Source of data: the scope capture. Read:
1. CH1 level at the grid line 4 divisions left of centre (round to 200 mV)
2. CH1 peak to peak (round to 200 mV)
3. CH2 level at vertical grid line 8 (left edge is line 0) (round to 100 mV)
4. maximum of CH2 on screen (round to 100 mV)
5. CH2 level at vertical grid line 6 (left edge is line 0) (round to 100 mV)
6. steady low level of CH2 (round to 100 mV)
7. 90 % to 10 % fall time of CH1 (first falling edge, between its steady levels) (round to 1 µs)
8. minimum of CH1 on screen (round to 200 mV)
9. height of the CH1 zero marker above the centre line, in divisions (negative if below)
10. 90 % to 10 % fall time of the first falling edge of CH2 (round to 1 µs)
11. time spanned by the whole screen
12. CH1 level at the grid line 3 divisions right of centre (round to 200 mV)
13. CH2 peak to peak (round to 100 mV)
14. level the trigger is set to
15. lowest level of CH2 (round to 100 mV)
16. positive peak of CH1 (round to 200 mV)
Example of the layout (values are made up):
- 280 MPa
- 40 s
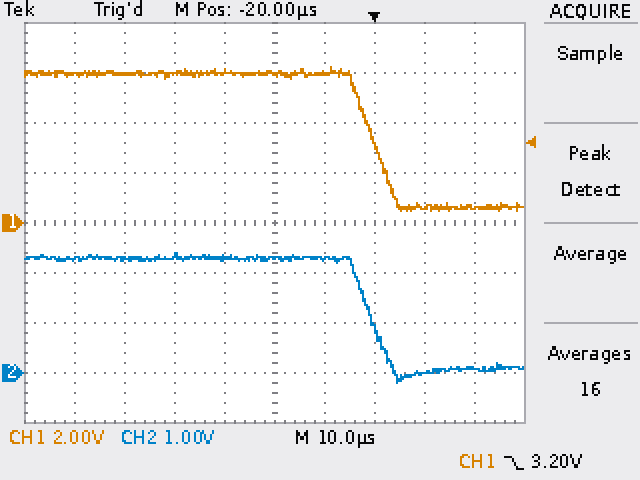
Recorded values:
- 6.0 V
- 5.8 V
- 0.0 V
- 2.4 V
- 2.3 V
- 100 mV
- 8 µs
- 400 mV
- 0.0 div
- 7 µs
- 100 µs
- 600 mV
- 2.6 V
- 3.20 V
- -200 mV
- 6.2 V
